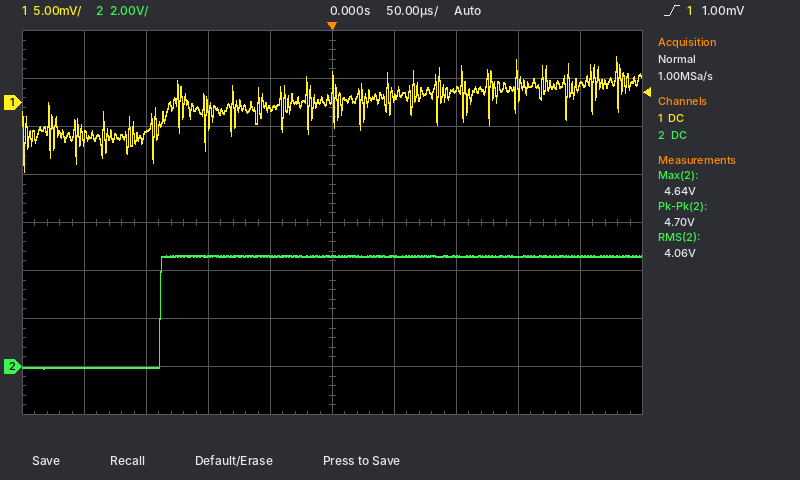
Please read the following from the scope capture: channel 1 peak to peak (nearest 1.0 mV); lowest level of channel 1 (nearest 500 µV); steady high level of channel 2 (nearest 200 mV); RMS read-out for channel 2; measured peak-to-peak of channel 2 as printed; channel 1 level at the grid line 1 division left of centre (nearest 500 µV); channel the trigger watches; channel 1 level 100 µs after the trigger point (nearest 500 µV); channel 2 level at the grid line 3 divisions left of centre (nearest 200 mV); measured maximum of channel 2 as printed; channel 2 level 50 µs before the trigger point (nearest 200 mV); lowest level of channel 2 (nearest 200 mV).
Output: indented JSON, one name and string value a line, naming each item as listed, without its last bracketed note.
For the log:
{
  "channel 1 peak to peak": "12.0 mV",
  "lowest level of channel 1": "-7.0 mV",
  "steady high level of channel 2": "4.6 V",
  "RMS read-out for channel 2": "4.06 V",
  "measured peak-to-peak of channel 2 as printed": "4.70 V",
  "channel 1 level at the grid line 1 division left of centre": "-500 µV",
  "channel the trigger watches": "channel 1",
  "channel 1 level 100 µs after the trigger point": "1.5 mV",
  "channel 2 level at the grid line 3 divisions left of centre": "0.0 V",
  "measured maximum of channel 2 as printed": "4.64 V",
  "channel 2 level 50 µs before the trigger point": "4.6 V",
  "lowest level of channel 2": "0.0 V"
}
